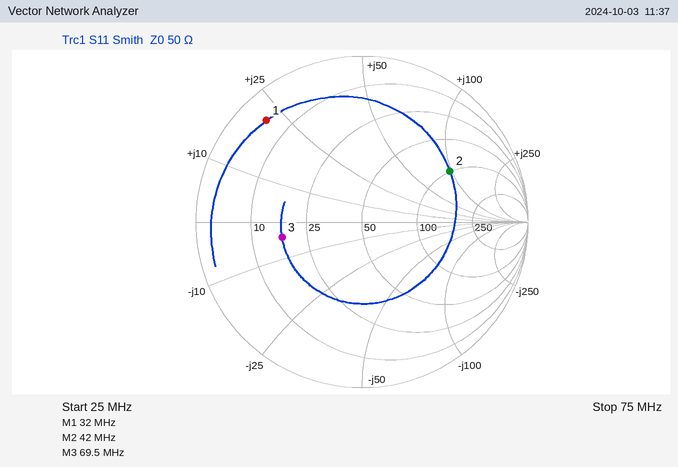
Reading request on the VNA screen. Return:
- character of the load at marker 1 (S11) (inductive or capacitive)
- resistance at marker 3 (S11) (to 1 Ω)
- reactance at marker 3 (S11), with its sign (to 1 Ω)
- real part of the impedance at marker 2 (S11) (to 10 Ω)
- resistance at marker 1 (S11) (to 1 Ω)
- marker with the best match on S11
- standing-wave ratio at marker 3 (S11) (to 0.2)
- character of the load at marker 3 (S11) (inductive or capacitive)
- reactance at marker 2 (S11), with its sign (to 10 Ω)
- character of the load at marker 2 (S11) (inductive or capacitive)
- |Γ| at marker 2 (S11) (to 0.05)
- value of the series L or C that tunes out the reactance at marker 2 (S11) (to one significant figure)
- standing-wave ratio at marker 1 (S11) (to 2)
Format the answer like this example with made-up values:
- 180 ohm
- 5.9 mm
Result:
- inductive
- 17 Ω
- -4 Ω
- 100 Ω
- 5 Ω
- marker 3
- 3.0
- capacitive
- +100 Ω
- inductive
- 0.60
- 40 pF
- 12
